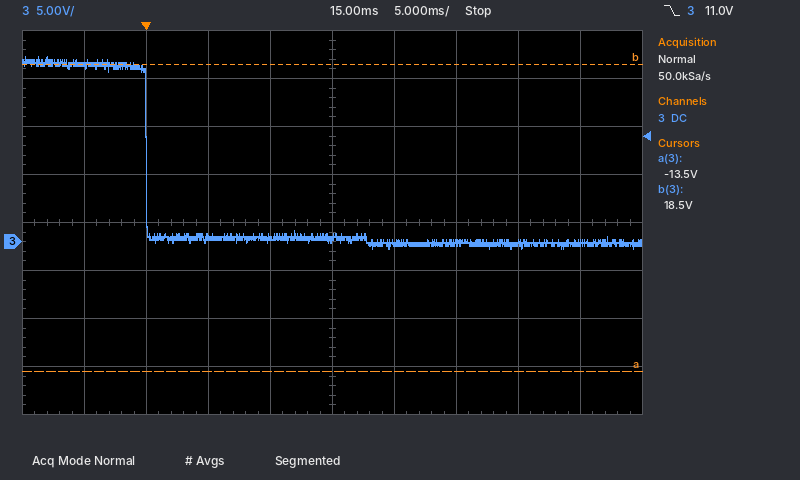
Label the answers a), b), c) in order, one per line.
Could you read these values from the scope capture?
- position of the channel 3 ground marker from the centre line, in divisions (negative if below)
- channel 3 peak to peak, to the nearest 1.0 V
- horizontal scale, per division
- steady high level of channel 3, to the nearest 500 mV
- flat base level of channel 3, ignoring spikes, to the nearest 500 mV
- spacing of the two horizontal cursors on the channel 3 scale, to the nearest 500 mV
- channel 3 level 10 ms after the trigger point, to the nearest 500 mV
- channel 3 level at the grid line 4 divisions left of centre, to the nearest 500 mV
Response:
a) -0.4 div
b) 20.0 V
c) 5 ms
d) 18.5 V
e) 0.0 V
f) 32.0 V
g) 500 mV
h) 18.5 V
